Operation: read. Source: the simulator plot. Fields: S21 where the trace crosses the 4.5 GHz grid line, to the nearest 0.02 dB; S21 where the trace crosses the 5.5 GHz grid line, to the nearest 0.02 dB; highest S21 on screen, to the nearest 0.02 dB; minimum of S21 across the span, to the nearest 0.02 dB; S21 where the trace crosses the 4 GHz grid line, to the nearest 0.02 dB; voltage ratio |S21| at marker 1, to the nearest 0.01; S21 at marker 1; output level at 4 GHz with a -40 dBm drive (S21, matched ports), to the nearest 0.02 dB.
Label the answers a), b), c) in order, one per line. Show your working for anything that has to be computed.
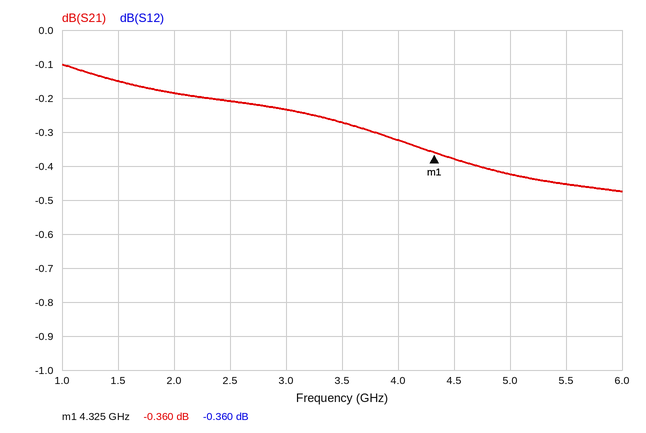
a) -0.38 dB
b) -0.46 dB
c) -0.10 dB
d) -0.48 dB
e) -0.32 dB
f) 10^(-0.36/20) ≈ 0.96
g) -0.360 dB
h) -40 dBm + (-0.32 dB) = -40.32 dBm
